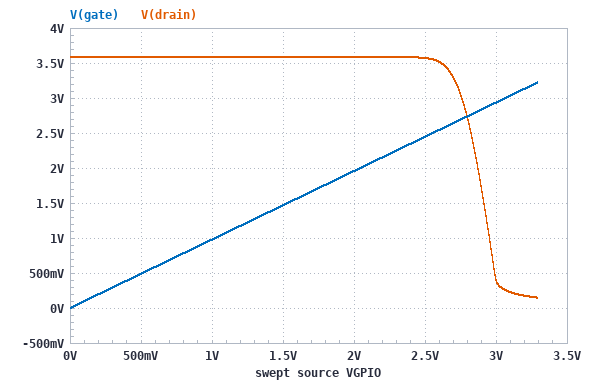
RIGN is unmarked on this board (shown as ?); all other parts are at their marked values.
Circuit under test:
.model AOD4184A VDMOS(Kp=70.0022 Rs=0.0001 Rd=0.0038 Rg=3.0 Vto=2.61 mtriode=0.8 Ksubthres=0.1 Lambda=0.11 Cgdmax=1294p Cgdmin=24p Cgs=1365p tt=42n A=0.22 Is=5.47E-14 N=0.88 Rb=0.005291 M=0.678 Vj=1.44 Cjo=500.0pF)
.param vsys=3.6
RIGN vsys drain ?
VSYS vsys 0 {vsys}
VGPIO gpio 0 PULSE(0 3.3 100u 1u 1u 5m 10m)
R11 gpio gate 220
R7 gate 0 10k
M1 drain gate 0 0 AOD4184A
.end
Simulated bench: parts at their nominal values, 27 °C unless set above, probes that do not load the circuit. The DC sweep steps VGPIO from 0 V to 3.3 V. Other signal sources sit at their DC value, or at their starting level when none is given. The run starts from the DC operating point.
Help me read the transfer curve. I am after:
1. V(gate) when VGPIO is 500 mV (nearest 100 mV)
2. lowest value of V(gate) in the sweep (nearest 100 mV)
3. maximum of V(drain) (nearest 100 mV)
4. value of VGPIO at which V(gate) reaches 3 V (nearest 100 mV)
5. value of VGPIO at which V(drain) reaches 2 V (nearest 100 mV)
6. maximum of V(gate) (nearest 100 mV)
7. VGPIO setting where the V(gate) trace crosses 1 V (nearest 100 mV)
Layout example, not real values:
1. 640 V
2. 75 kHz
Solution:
1. 500 mV
2. 0 V
3. 3.6 V
4. 3.1 V
5. 2.9 V
6. 3.2 V
7. 1.0 V
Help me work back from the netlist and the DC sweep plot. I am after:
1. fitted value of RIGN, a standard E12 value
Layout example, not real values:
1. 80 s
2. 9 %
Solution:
1. 0.82 Ω
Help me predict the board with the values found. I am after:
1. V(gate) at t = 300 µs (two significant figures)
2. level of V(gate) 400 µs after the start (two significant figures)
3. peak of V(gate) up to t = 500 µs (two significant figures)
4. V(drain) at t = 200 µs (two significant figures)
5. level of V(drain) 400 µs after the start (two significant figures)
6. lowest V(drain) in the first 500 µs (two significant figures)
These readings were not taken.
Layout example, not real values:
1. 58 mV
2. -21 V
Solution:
1. 3.2 V
2. 3.2 V
3. 3.2 V
4. 150 mV
5. 150 mV
6. 150 mV
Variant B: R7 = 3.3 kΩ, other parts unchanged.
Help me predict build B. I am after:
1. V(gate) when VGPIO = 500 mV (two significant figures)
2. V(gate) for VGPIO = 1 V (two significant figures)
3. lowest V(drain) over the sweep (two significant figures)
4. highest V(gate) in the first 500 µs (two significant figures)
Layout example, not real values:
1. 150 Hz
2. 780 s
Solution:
1. 470 mV
2. 940 mV
3. 190 mV
4. 3.1 V
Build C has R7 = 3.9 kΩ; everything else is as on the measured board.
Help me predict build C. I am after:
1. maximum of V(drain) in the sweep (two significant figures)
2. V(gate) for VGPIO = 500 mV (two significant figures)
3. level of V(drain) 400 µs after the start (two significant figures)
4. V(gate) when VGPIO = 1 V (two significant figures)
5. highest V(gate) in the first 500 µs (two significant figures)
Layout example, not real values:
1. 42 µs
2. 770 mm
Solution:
1. 3.6 V
2. 470 mV
3. 180 mV
4. 950 mV
5. 3.1 V
